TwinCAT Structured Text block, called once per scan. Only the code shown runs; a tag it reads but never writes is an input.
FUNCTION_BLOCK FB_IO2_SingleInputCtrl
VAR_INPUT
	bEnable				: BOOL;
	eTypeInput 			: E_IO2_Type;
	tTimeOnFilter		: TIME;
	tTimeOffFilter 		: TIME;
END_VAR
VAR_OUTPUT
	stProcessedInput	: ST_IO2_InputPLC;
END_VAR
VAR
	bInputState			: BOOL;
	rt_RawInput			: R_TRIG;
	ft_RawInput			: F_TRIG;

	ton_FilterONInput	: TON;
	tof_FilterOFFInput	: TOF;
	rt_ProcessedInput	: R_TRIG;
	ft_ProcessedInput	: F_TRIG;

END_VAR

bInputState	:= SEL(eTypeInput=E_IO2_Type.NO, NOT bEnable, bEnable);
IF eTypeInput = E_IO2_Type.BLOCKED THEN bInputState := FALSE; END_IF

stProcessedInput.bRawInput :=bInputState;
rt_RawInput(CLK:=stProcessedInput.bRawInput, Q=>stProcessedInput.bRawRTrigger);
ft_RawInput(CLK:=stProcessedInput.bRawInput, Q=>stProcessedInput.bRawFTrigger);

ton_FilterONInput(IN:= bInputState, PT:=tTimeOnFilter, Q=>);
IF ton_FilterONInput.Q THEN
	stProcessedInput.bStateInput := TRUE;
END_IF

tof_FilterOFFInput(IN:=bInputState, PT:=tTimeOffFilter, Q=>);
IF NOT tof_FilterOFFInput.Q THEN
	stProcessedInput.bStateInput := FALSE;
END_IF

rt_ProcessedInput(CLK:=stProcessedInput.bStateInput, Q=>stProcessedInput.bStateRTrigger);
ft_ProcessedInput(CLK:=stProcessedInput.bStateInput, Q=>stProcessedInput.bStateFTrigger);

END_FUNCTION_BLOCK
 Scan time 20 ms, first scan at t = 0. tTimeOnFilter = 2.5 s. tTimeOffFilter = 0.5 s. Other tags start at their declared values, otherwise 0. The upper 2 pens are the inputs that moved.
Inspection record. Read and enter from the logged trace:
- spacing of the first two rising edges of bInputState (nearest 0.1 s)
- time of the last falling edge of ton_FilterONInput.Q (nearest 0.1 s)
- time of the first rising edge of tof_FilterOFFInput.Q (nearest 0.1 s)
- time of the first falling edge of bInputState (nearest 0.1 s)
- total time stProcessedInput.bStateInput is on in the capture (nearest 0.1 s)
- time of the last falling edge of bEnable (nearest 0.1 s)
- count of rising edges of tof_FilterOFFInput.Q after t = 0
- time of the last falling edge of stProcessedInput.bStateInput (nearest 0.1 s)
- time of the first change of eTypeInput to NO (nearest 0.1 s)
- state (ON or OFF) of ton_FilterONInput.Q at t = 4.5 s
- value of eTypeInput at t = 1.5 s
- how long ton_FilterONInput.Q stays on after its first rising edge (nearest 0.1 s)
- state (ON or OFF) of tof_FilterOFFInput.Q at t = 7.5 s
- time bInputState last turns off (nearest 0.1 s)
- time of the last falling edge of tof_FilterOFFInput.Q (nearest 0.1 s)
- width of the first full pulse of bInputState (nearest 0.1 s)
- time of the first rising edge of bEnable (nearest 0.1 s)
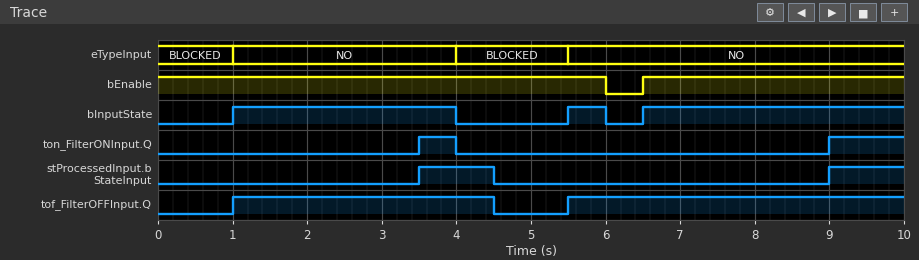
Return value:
4.5 s
4.0 s
1.0 s
4.0 s
2.0 s
6.0 s
2
4.5 s
1.0 s
OFF
NO
0.5 s
ON
6.0 s
4.5 s
3.0 s
6.5 s
